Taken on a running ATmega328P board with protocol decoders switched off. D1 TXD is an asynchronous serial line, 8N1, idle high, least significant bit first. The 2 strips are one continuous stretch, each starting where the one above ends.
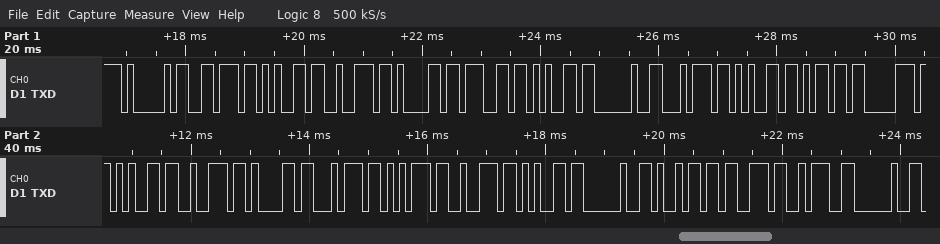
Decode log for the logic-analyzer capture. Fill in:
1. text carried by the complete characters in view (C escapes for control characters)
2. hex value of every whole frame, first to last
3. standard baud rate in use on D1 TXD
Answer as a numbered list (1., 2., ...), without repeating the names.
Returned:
1. "Average temperature is: "
2. 41 76 65 72 61 67 65 20 74 65 6D 70 65 72 61 74 75 72 65 20 69 73 3A 20
3. 9600 baud
